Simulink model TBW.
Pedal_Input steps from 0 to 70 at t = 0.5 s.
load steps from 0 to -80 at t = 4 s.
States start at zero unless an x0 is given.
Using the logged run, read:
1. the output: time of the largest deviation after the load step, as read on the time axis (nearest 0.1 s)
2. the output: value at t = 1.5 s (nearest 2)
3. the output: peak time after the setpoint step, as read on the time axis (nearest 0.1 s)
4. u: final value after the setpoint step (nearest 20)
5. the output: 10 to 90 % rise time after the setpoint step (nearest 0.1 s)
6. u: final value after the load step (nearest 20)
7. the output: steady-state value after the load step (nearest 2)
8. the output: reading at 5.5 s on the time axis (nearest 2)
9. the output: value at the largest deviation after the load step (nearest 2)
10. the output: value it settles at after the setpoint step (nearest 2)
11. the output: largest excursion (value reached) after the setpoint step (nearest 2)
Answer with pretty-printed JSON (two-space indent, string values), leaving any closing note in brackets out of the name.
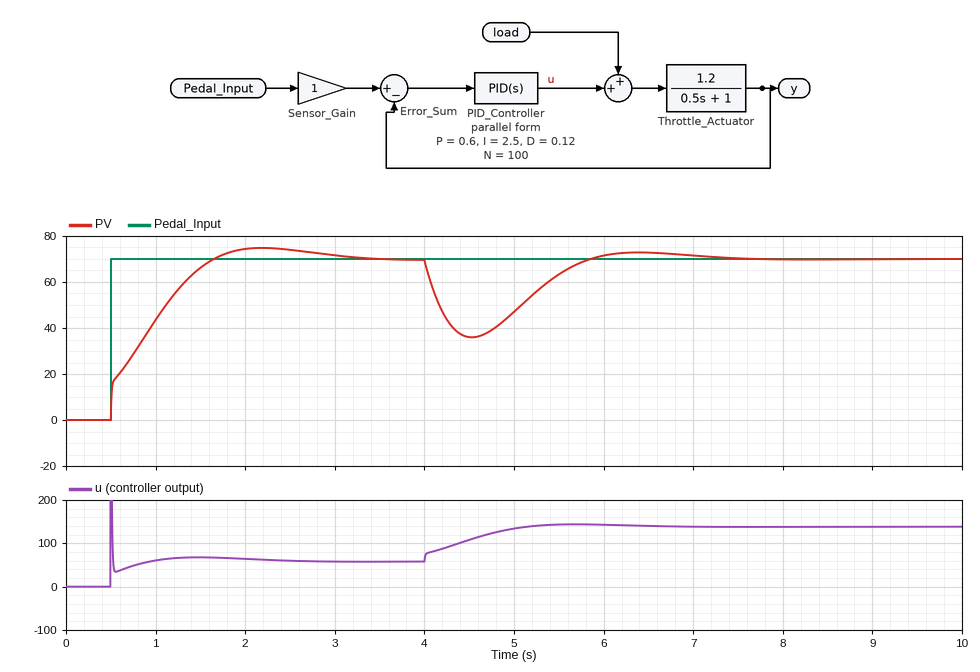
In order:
{
  "the output: time of the largest deviation after the load step, as read on the time axis": "4.5 s",
  "the output: value at t = 1.5 s": "66",
  "the output: peak time after the setpoint step, as read on the time axis": "2.2 s",
  "u: final value after the setpoint step": "60",
  "the output: 10 to 90 % rise time after the setpoint step": "0.9 s",
  "u: final value after the load step": "140",
  "the output: steady-state value after the load step": "70",
  "the output: reading at 5.5 s on the time axis": "64",
  "the output: value at the largest deviation after the load step": "36",
  "the output: value it settles at after the setpoint step": "70",
  "the output: largest excursion (value reached) after the setpoint step": "74"
}
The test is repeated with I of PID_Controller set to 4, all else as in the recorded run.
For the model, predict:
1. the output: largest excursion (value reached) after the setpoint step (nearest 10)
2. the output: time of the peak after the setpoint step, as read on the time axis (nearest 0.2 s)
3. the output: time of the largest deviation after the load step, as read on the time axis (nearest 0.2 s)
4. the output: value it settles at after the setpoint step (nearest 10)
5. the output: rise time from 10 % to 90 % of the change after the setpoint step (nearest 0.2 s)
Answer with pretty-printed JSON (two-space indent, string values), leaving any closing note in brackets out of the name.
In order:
{
  "the output: largest excursion (value reached) after the setpoint step": "80",
  "the output: time of the peak after the setpoint step, as read on the time axis": "1.8 s",
  "the output: time of the largest deviation after the load step, as read on the time axis": "4.4 s",
  "the output: value it settles at after the setpoint step": "70",
  "the output: rise time from 10 % to 90 % of the change after the setpoint step": "0.6 s"
}
